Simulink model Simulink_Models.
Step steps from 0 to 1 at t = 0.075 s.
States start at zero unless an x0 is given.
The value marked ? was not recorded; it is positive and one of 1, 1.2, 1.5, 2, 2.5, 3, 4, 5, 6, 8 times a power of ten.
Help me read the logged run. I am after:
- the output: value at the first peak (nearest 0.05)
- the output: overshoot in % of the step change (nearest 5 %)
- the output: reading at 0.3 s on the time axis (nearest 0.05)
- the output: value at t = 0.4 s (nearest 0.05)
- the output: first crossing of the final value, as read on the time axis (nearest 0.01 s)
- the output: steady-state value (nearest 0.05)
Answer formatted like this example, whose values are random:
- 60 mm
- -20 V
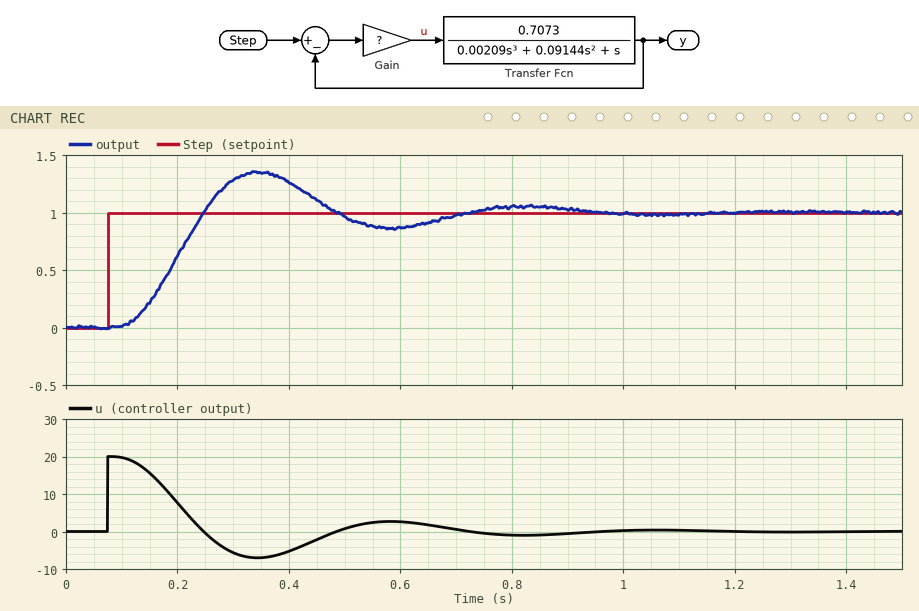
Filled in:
- 1.35
- 35 %
- 1.30
- 1.25
- 0.25 s
- 1.00
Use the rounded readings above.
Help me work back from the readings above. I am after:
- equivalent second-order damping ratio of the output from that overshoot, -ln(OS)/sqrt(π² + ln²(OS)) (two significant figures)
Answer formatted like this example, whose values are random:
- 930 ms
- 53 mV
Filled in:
- 0.32
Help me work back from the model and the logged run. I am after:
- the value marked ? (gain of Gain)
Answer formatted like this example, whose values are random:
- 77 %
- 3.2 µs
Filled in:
- 20
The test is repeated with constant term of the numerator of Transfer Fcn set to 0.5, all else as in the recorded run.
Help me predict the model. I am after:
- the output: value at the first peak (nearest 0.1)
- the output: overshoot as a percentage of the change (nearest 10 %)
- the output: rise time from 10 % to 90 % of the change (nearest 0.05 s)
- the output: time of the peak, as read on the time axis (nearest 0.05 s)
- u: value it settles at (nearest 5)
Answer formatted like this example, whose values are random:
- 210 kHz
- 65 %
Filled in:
- 1.2
- 20 %
- 0.15 s
- 0.40 s
- 0
